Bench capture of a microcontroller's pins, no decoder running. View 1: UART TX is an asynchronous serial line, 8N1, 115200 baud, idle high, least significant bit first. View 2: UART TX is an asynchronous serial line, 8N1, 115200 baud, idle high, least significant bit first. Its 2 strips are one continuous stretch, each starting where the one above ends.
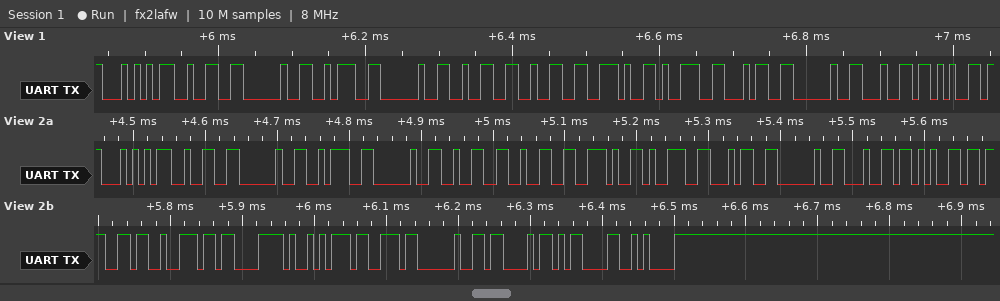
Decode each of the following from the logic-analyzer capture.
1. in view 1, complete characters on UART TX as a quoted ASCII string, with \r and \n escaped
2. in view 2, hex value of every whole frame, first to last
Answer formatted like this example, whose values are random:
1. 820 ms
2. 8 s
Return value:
1. "T2 : 22.94 de"
2. 0x54 0x32 0x20 0x3A 0x20 0x32 0x32 0x2E 0x39 0x34 0x20 0x64 0x65 0x67 0x72 0xC3 0xA9 0x73 0x20 0x43 0x0D 0x0A
